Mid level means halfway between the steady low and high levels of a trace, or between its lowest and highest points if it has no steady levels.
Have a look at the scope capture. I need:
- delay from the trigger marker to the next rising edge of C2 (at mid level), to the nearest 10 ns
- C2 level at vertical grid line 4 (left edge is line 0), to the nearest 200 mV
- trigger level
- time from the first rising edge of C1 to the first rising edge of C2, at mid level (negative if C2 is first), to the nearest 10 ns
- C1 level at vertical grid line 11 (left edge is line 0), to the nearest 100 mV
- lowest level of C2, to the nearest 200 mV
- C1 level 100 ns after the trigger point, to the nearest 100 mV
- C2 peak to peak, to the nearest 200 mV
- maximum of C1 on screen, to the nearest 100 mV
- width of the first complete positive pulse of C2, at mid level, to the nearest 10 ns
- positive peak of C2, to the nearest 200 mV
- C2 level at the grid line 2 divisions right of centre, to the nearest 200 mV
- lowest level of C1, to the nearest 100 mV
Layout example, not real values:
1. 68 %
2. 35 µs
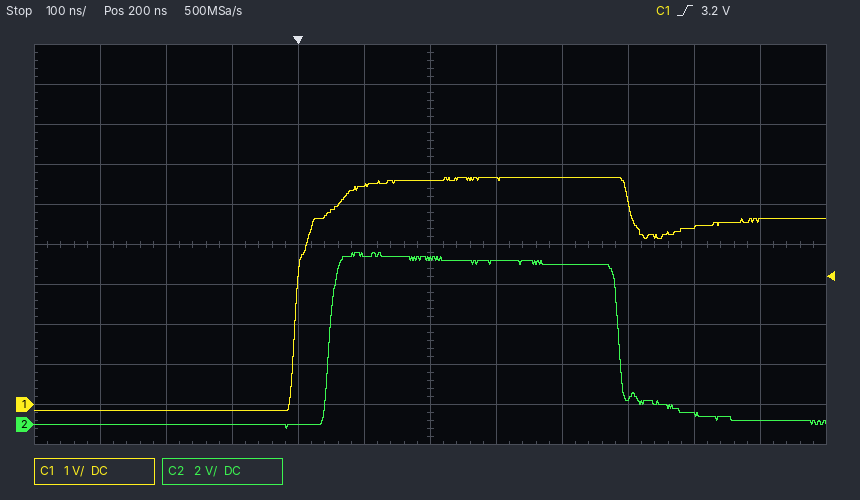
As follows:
1. 50 ns
2. 0.0 V
3. 3.2 V
4. +50 ns
5. 4.6 V
6. -200 mV
7. 5.5 V
8. 8.8 V
9. 5.7 V
10. 440 ns
11. 8.6 V
12. 8.0 V
13. -200 mV
